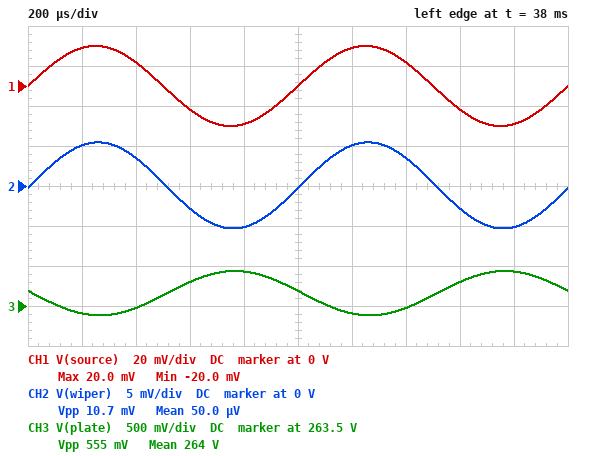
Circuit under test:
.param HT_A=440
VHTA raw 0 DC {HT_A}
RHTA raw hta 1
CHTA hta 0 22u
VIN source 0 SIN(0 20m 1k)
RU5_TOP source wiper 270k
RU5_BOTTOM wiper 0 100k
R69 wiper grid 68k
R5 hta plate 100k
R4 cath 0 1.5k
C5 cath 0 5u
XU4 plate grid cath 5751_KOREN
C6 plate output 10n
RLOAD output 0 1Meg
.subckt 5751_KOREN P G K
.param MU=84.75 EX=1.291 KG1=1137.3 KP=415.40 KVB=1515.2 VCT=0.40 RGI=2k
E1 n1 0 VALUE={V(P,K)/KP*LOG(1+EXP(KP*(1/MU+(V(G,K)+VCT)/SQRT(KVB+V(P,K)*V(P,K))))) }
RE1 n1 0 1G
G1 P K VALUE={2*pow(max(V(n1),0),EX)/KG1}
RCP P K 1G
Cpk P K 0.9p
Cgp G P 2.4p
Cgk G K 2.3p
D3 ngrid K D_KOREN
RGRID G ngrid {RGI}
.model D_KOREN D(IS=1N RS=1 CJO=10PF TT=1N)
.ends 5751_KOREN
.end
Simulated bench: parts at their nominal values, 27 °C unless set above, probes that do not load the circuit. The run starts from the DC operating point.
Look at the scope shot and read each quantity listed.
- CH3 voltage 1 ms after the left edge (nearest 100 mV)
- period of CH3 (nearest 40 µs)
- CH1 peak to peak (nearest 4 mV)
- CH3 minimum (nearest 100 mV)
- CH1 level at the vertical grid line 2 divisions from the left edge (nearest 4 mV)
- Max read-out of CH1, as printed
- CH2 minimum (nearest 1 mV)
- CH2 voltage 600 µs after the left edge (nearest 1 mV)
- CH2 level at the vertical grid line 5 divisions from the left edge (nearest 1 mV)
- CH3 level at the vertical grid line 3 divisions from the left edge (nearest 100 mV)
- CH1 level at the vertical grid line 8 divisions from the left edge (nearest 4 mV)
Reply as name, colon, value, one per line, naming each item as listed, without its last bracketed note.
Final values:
CH3 voltage 1 ms after the left edge: 263.7 V
period of CH3: 1.00 ms
CH1 peak to peak: 40 mV
CH3 minimum: 263.4 V
CH1 level at the vertical grid line 2 divisions from the left edge: 12 mV
Max read-out of CH1, as printed: 20.0 mV
CH2 minimum: -5 mV
CH2 voltage 600 µs after the left edge: -3 mV
CH2 level at the vertical grid line 5 divisions from the left edge: 0 V
CH3 level at the vertical grid line 3 divisions from the left edge: 263.8 V
CH1 level at the vertical grid line 8 divisions from the left edge: -12 mV
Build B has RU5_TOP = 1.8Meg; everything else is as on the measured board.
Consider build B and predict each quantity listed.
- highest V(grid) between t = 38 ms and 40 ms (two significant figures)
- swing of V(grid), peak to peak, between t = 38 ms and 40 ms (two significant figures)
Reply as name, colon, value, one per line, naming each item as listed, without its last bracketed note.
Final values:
highest V(grid) between t = 38 ms and 40 ms: 1.2 mV
swing of V(grid), peak to peak, between t = 38 ms and 40 ms: 2.1 mV
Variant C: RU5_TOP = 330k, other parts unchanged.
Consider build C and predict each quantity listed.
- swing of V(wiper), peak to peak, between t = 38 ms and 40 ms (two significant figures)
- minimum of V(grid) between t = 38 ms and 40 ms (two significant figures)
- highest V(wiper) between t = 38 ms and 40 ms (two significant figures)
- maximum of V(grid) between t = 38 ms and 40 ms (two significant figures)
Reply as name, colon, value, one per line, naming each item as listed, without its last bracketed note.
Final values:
swing of V(wiper), peak to peak, between t = 38 ms and 40 ms: 9.3 mV
minimum of V(grid) between t = 38 ms and 40 ms: -4.5 mV
highest V(wiper) between t = 38 ms and 40 ms: 4.7 mV
maximum of V(grid) between t = 38 ms and 40 ms: 4.8 mV
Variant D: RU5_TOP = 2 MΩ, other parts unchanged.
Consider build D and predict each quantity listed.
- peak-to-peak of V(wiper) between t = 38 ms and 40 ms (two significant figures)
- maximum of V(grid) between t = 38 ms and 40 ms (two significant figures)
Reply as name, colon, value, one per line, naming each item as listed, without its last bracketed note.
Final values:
peak-to-peak of V(wiper) between t = 38 ms and 40 ms: 1.9 mV
maximum of V(grid) between t = 38 ms and 40 ms: 1.1 mV
